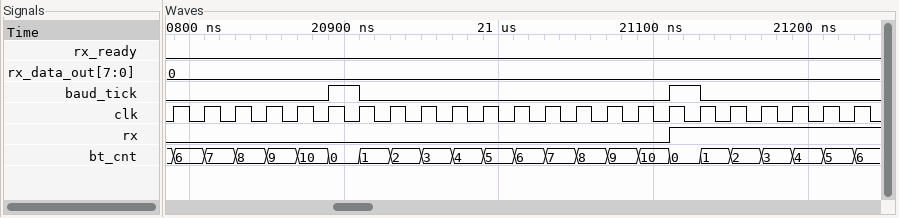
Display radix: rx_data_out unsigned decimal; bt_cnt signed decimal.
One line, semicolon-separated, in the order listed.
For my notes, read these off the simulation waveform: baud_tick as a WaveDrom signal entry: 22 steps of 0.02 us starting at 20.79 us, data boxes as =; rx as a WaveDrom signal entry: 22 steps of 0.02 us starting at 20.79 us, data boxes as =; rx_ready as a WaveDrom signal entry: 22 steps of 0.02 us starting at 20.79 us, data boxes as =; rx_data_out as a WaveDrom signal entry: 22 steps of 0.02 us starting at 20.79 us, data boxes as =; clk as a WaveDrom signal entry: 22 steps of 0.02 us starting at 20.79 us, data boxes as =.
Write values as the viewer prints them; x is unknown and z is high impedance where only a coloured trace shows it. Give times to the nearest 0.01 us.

{name: 'baud_tick', wave: '0....10.........10....'}; {name: 'rx', wave: '0...............1.....'}; {name: 'rx_ready', wave: '0.....................'}; {name: 'rx_data_out', wave: '=.....................', data: '0'}; {name: 'clk', wave: 'p.....................'}
